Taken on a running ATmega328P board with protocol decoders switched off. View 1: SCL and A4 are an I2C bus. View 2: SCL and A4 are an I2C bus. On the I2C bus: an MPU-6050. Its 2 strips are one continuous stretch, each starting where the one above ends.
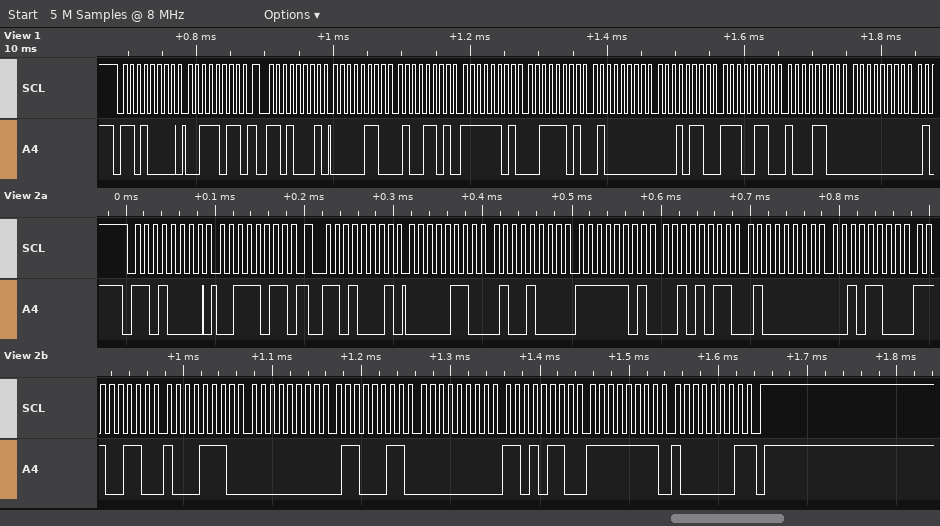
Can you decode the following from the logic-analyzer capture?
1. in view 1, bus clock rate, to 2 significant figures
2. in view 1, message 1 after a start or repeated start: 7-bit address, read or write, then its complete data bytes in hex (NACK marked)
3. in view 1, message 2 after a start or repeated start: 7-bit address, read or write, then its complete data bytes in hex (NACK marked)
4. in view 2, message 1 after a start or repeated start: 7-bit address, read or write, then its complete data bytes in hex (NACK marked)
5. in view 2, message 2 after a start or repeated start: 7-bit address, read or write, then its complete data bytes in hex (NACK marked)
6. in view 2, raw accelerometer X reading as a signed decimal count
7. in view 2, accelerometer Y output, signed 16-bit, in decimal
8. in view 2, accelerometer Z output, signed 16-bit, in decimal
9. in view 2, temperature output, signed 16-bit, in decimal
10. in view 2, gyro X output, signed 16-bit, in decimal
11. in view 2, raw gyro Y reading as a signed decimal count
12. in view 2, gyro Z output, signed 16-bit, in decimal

100 kHz
0x68 write: 3B
0x68 read: 06 4D FD 3D 40 16 E6 8C 00
0x68 write: 3B
0x68 read: 06 48 FD 2B 40 2C E6 8E 00 63 00 D6 FF 81 NACK
1608
-725
16428
-6514
99
214
-127
